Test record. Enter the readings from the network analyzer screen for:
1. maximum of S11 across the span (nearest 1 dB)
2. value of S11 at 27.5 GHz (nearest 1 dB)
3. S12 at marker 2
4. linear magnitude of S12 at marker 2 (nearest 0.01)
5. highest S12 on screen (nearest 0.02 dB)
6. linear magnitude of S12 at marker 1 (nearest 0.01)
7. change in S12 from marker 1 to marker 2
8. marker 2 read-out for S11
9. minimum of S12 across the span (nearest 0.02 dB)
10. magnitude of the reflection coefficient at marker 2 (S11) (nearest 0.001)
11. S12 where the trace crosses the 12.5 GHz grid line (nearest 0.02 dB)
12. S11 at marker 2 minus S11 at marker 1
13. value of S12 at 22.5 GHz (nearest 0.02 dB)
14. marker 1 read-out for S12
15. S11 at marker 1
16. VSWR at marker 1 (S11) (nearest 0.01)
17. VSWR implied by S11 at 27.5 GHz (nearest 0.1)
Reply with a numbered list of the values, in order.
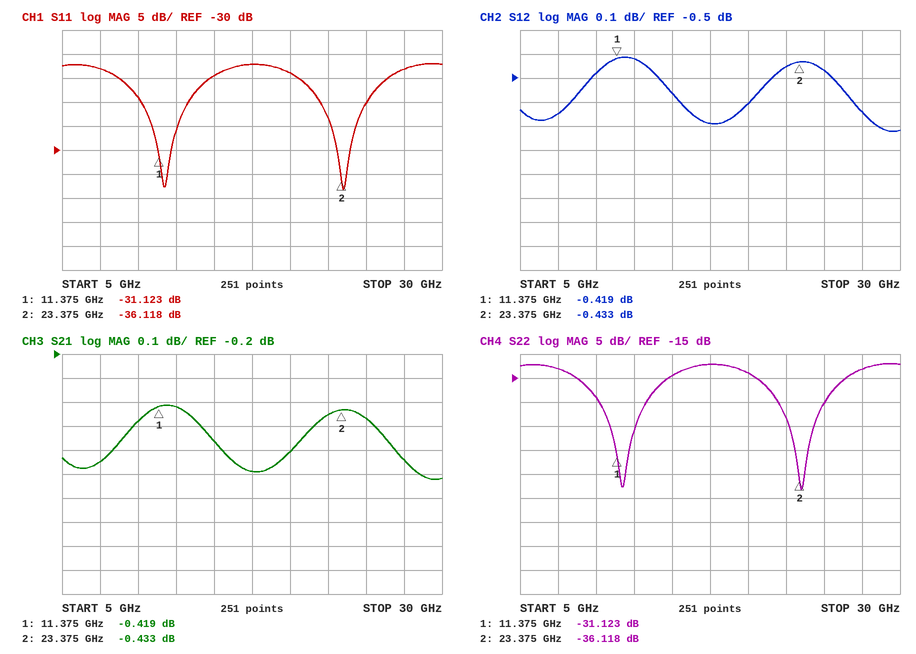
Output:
1. -12 dB
2. -13 dB
3. -0.433 dB
4. 0.95
5. -0.42 dB
6. 0.95
7. -0.014 dB
8. -36.118 dB
9. -0.72 dB
10. 0.016
11. -0.42 dB
12. -4.995 dB
13. -0.46 dB
14. -0.419 dB
15. -31.123 dB
16. 1.06
17. 1.6
